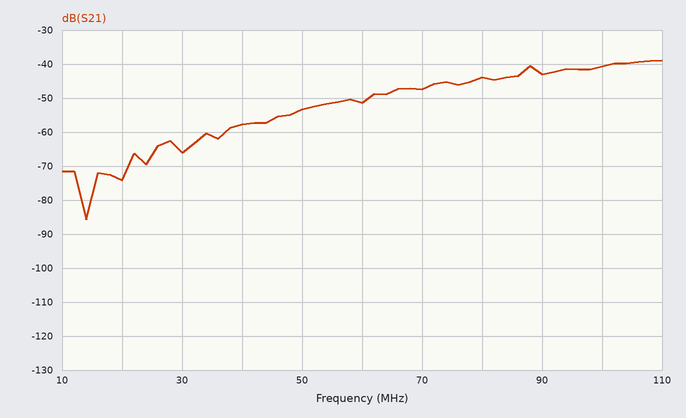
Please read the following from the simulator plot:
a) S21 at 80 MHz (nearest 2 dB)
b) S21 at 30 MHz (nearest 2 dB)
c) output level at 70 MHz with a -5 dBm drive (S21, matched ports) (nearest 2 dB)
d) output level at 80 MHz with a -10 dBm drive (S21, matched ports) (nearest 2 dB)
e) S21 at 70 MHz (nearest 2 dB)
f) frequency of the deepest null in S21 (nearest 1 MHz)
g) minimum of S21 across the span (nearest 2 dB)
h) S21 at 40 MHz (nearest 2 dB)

-44 dB
-66 dB
-52 dBm
-54 dBm
-48 dB
14 MHz
-86 dB
-58 dB
